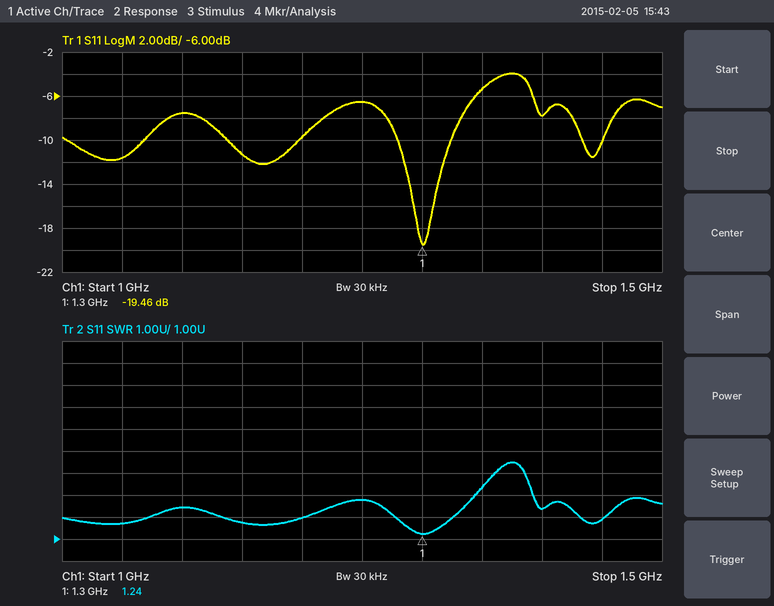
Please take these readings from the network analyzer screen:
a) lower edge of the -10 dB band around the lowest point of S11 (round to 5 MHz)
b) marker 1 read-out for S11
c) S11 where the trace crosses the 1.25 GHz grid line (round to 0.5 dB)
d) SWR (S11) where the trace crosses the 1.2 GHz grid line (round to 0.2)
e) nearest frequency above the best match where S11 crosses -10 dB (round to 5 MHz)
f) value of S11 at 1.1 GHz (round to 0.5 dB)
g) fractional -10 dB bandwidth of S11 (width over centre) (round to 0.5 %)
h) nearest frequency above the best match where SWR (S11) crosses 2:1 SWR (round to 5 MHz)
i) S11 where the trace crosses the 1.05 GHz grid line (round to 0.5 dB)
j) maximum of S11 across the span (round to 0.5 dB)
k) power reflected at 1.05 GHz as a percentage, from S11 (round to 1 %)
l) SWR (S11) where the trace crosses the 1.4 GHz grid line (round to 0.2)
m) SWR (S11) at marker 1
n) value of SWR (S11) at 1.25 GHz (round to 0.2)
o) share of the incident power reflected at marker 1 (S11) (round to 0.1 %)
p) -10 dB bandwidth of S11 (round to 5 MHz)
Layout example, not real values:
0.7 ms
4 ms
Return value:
1.280 GHz
-19.46 dB
-6.5 dB
2.0
1.325 GHz
-7.5 dB
3.5 %
1.325 GHz
-11.5 dB
-4.0 dB
7 %
2.4
1.24
2.8
1.1 %
45 MHz
